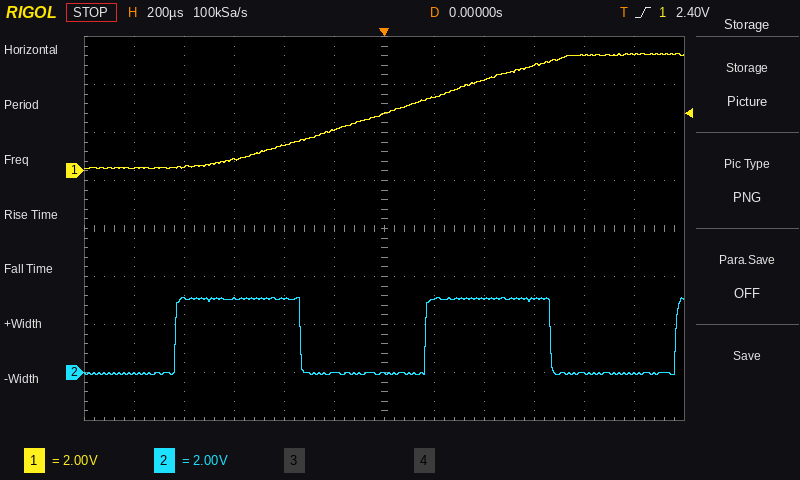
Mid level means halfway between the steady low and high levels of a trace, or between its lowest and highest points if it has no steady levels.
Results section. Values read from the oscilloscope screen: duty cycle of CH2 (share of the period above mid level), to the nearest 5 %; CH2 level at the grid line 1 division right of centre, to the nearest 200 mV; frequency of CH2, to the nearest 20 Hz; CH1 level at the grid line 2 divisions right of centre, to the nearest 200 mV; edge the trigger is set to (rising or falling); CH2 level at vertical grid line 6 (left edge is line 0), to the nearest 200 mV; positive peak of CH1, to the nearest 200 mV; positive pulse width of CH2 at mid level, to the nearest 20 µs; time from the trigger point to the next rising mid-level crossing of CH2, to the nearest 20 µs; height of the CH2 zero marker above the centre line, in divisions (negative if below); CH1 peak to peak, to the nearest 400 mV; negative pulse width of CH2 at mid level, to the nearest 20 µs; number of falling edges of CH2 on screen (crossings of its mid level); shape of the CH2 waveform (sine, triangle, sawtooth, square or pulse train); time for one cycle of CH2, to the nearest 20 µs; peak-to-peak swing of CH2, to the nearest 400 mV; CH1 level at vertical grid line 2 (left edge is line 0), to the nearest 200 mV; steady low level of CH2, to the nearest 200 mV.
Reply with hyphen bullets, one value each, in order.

- 50 %
- 3.0 V
- 1.00 kHz
- 3.8 V
- rising
- 0.0 V
- 4.8 V
- 500 µs
- 160 µs
- -3.0 div
- 4.8 V
- 500 µs
- 2
- square
- 1.00 ms
- 3.2 V
- 200 mV
- 0.0 V
